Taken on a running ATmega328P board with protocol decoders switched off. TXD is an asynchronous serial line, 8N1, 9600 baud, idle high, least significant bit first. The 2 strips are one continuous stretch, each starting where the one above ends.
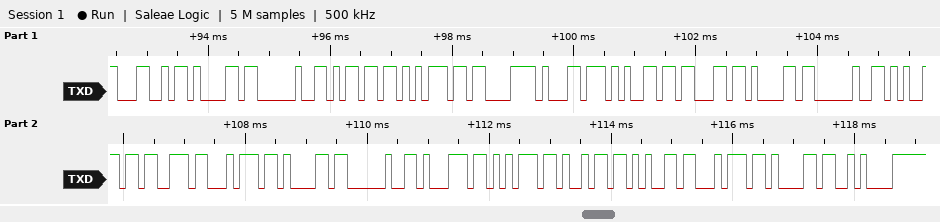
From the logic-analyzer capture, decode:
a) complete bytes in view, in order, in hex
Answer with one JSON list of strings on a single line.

["0x4C 0x61 0x20 0x6D 0x75 0xC3 0xB1 0x65 0x63 0x61 0x20 0x65 0x73 0x74 0x61 0x20 0x71 0x75 0x69 0x65 0x74 0x61 0x0A"]
